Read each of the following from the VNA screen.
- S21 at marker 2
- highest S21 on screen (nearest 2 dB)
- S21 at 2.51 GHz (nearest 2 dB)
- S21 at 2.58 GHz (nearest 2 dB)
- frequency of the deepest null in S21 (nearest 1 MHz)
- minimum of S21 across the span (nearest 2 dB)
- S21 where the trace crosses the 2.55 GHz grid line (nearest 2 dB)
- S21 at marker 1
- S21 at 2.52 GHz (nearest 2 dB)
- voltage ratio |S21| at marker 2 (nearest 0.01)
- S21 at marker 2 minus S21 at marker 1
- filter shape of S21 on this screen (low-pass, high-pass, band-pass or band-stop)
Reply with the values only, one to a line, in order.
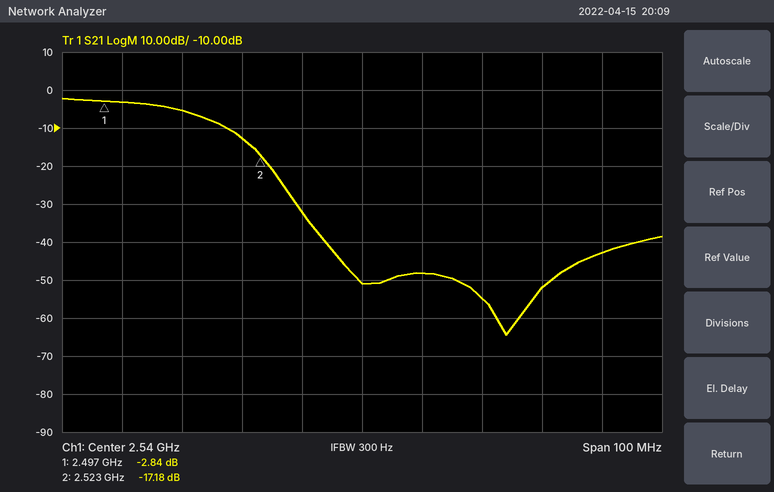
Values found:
-17.18 dB
-2 dB
-6 dB
-42 dB
2.564 GHz
-64 dB
-48 dB
-2.84 dB
-12 dB
0.14
-14.34 dB
low-pass
